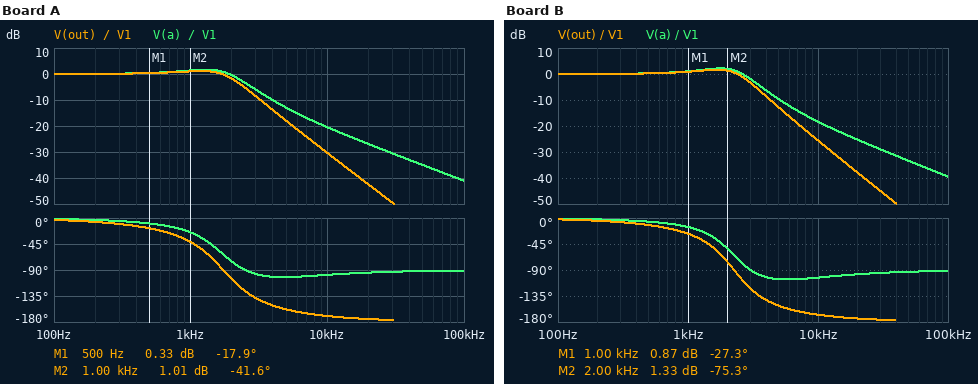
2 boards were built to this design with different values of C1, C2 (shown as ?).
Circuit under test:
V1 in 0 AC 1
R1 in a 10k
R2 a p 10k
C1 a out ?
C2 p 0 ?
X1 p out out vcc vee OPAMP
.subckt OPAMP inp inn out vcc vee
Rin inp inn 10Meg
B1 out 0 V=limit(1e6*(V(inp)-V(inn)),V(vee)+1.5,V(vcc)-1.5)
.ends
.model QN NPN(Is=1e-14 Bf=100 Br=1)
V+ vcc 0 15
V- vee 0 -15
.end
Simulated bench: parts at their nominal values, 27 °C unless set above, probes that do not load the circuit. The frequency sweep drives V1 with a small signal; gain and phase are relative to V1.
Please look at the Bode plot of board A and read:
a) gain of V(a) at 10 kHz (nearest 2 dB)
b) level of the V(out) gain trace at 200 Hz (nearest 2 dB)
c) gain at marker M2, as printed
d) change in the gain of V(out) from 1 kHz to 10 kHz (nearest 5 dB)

-20 dB
0 dB
1.01 dB
-30 dB
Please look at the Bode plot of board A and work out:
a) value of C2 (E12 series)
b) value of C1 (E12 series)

4.7 nF
18 nF
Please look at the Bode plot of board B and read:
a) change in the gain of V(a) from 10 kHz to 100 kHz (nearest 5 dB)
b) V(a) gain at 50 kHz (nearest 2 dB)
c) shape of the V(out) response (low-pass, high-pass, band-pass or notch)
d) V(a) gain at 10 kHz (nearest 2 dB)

-20 dB
-34 dB
low-pass
-18 dB
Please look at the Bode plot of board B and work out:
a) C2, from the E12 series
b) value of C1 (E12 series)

3.3 nF
15 nF
